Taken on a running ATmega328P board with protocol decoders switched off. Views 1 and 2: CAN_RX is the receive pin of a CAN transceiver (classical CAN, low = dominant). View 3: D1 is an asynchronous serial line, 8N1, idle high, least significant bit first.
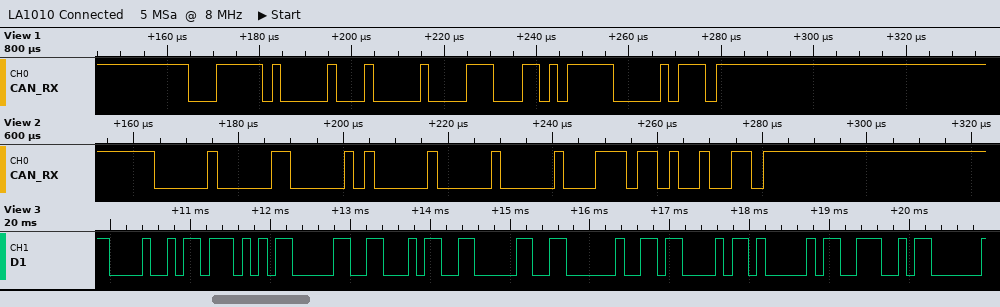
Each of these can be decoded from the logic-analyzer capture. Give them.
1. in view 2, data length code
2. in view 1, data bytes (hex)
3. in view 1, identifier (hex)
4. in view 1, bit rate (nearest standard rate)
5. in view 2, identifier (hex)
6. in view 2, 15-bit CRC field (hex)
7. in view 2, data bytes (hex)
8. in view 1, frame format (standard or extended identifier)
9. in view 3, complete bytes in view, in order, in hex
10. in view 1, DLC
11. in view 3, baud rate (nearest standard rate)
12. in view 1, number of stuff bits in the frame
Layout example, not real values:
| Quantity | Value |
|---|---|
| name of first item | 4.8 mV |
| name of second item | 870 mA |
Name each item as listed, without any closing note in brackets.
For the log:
| Quantity | Value |
|---|---|
| in view 2, data length code | 2 |
| in view 1, data bytes | 00 E3 |
| in view 1, identifier | 0x1F8 |
| in view 1, bit rate | 500 kbit/s |
| in view 2, identifier | 0x002 |
| in view 2, 15-bit CRC field | 0x3B49 |
| in view 2, data bytes | 00 00 |
| in view 1, frame format | standard |
| in view 3, complete bytes in view, in order, in hex | 0x48 0x57 0x30 0x34 0x30 0x20 0x43 0x41 0x4E |
| in view 1, DLC | 2 |
| in view 3, baud rate | 9600 baud |
| in view 1, number of stuff bits in the frame | 5 |
